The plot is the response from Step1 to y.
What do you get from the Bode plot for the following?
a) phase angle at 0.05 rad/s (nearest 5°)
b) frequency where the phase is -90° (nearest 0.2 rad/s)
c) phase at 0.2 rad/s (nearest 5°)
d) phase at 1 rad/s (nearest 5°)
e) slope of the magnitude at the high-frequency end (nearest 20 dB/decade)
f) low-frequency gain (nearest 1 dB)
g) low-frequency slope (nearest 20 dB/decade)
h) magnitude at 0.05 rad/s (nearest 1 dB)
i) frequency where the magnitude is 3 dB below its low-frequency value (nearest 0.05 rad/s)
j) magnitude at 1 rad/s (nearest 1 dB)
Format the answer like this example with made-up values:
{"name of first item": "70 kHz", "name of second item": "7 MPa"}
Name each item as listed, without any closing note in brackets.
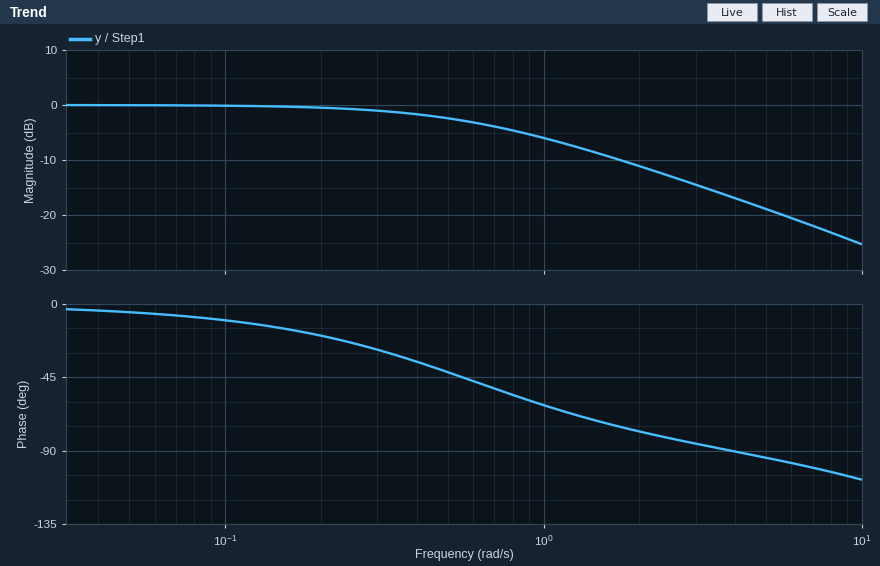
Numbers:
{"phase angle at 0.05 rad/s": "-5°", "frequency where the phase is -90°": "3.8 rad/s", "phase at 0.2 rad/s": "-20°", "phase at 1 rad/s": "-60°", "slope of the magnitude at the high-frequency end": "-20 dB/decade", "low-frequency gain": "0 dB", "low-frequency slope": "0 dB/decade", "magnitude at 0.05 rad/s": "0 dB", "frequency where the magnitude is 3 dB below its low-frequency value": "0.60 rad/s", "magnitude at 1 rad/s": "-6 dB"}
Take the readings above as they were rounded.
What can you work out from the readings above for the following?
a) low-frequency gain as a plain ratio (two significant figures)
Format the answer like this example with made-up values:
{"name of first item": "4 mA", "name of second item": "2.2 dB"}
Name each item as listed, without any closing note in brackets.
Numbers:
{"low-frequency gain as a plain ratio": "1.0"}
